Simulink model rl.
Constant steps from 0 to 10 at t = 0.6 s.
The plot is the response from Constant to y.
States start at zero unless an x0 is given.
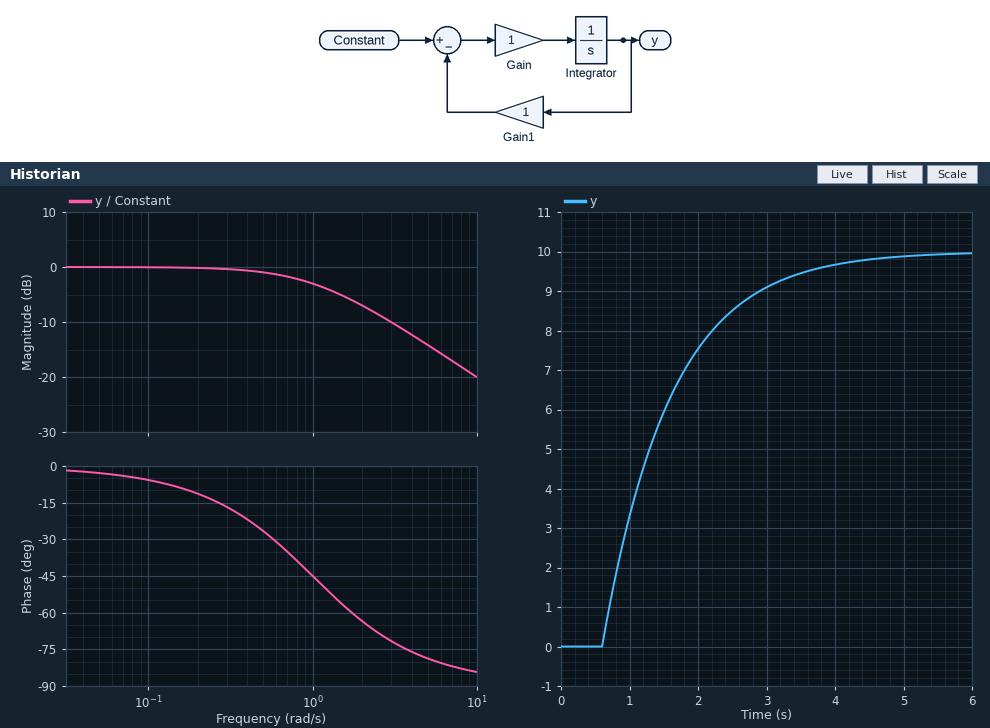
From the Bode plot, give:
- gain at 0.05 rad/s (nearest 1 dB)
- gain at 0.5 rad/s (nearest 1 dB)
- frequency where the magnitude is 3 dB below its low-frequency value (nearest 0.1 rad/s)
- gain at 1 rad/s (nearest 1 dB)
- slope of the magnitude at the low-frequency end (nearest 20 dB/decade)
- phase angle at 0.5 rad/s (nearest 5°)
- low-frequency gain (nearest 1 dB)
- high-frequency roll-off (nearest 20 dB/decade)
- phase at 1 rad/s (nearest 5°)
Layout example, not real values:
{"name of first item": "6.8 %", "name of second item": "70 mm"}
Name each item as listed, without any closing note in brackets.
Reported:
{"gain at 0.05 rad/s": "0 dB", "gain at 0.5 rad/s": "-1 dB", "frequency where the magnitude is 3 dB below its low-frequency value": "1.0 rad/s", "gain at 1 rad/s": "-3 dB", "slope of the magnitude at the low-frequency end": "0 dB/decade", "phase angle at 0.5 rad/s": "-25°", "low-frequency gain": "0 dB", "high-frequency roll-off": "-20 dB/decade", "phase at 1 rad/s": "-45°"}
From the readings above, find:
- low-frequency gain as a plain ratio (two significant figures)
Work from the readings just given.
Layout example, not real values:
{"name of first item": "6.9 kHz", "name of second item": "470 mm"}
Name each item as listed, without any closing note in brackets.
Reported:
{"low-frequency gain as a plain ratio": "1.0"}
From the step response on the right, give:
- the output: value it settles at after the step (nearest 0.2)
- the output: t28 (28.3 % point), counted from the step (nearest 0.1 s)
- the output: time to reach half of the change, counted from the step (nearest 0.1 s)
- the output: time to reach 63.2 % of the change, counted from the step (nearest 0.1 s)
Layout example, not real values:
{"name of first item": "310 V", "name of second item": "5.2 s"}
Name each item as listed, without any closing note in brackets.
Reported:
{"the output: value it settles at after the step": "10.0", "the output: t28 (28.3 % point), counted from the step": "0.3 s", "the output: time to reach half of the change, counted from the step": "0.7 s", "the output: time to reach 63.2 % of the change, counted from the step": "1.0 s"}
